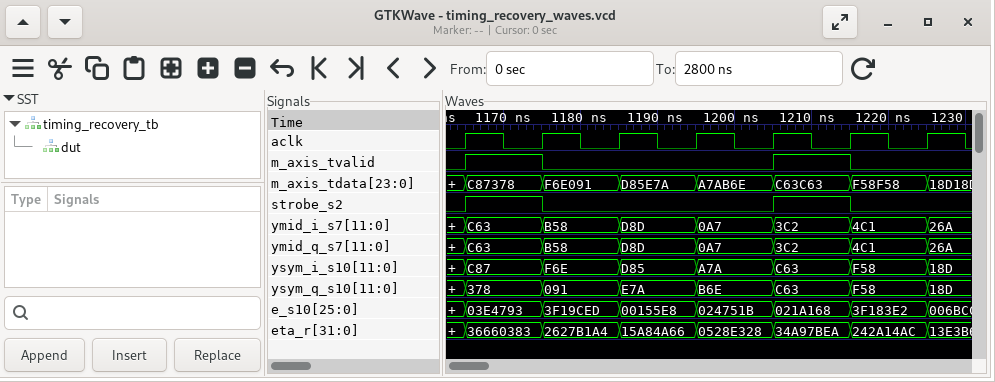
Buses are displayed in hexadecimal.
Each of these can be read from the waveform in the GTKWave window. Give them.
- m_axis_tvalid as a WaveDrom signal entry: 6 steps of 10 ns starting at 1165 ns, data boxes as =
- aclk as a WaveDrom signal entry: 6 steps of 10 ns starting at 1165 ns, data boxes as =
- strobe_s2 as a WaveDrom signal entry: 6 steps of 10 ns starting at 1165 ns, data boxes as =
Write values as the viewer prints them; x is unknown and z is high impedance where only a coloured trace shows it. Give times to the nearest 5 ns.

{name: 'm_axis_tvalid', wave: '10..10'}
{name: 'aclk', wave: 'p.....'}
{name: 'strobe_s2', wave: '10..10'}
